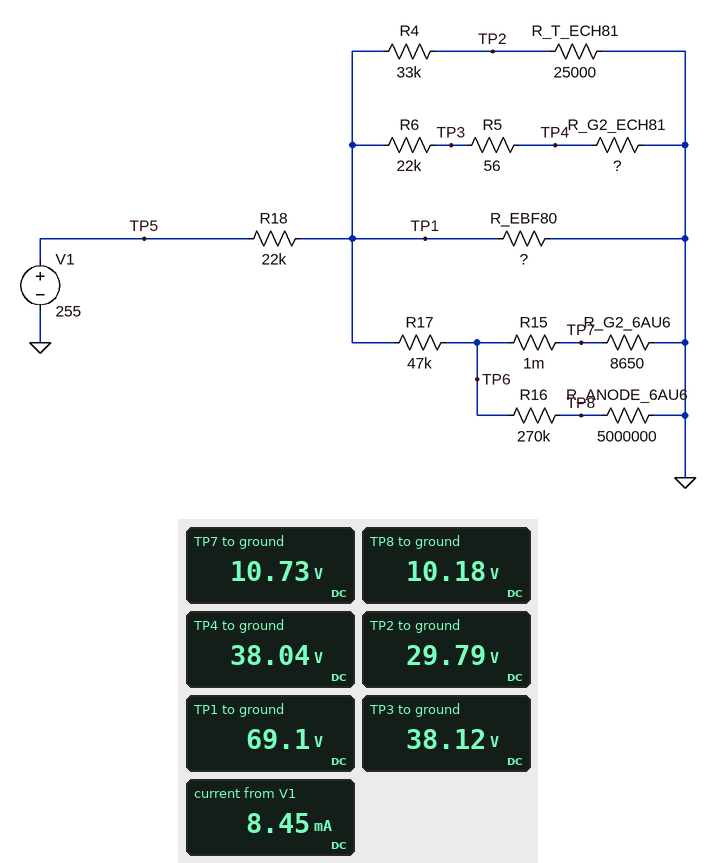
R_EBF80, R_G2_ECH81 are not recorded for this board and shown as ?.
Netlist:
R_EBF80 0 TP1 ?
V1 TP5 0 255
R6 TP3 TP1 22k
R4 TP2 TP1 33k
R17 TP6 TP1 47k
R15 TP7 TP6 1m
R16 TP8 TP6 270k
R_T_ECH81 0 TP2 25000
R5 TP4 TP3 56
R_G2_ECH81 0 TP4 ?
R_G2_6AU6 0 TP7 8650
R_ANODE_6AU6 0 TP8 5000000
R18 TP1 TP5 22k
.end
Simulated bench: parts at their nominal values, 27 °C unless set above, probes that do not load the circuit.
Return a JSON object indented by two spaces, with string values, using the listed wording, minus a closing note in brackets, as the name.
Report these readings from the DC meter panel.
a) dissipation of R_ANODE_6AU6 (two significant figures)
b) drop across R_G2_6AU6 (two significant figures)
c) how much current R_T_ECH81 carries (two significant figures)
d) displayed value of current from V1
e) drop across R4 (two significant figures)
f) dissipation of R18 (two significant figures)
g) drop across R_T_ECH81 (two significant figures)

{
  "dissipation of R_ANODE_6AU6": "21 µW",
  "drop across R_G2_6AU6": "11 V",
  "how much current R_T_ECH81 carries": "1.2 mA",
  "displayed value of current from V1": "8.45 mA",
  "drop across R4": "39 V",
  "dissipation of R18": "1.6 W",
  "drop across R_T_ECH81": "30 V"
}
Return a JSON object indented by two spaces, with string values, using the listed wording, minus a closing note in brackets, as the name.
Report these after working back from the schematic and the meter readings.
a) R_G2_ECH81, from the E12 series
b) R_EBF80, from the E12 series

{
  "R_G2_ECH81, from the E12 series": "27 kΩ",
  "R_EBF80, from the E12 series": "15 kΩ"
}
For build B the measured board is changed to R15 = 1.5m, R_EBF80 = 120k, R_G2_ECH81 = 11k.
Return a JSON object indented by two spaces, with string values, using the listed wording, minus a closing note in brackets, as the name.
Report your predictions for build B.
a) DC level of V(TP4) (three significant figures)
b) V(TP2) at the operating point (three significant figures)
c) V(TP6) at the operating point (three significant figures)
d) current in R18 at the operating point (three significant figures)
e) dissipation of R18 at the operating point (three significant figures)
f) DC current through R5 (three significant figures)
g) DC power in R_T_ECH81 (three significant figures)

{
  "DC level of V(TP4)": "32.3 V",
  "V(TP2) at the operating point": "41.9 V",
  "V(TP6) at the operating point": "15.1 V",
  "current in R18 at the operating point": "7.17 mA",
  "dissipation of R18 at the operating point": "1.13 W",
  "DC current through R5": "2.94 mA",
  "DC power in R_T_ECH81": "70.2 mW"
}
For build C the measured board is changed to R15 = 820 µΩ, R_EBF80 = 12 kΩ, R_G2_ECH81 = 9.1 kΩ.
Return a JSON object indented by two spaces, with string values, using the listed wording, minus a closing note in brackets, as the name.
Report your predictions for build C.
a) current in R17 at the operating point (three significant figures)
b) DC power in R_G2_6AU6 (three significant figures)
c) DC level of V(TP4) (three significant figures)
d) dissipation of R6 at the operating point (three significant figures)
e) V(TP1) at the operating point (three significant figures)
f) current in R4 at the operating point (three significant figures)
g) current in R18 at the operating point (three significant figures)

{
  "current in R17 at the operating point": "1.06 mA",
  "DC power in R_G2_6AU6": "9.73 mW",
  "DC level of V(TP4)": "17.3 V",
  "dissipation of R6 at the operating point": "79.2 mW",
  "V(TP1) at the operating point": "59.1 V",
  "current in R4 at the operating point": "1.02 mA",
  "current in R18 at the operating point": "8.90 mA"
}
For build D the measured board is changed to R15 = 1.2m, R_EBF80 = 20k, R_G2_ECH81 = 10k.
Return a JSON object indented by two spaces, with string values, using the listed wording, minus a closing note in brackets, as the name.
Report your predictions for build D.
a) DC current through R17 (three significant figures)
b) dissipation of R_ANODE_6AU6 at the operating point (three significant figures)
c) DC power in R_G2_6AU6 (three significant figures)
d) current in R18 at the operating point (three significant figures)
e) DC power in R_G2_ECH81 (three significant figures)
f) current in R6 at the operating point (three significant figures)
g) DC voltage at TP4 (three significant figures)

{
  "DC current through R17": "1.29 mA",
  "dissipation of R_ANODE_6AU6 at the operating point": "22.2 µW",
  "DC power in R_G2_6AU6": "14.3 mW",
  "current in R18 at the operating point": "8.34 mA",
  "DC power in R_G2_ECH81": "49.9 mW",
  "current in R6 at the operating point": "2.23 mA",
  "DC voltage at TP4": "22.3 V"
}
